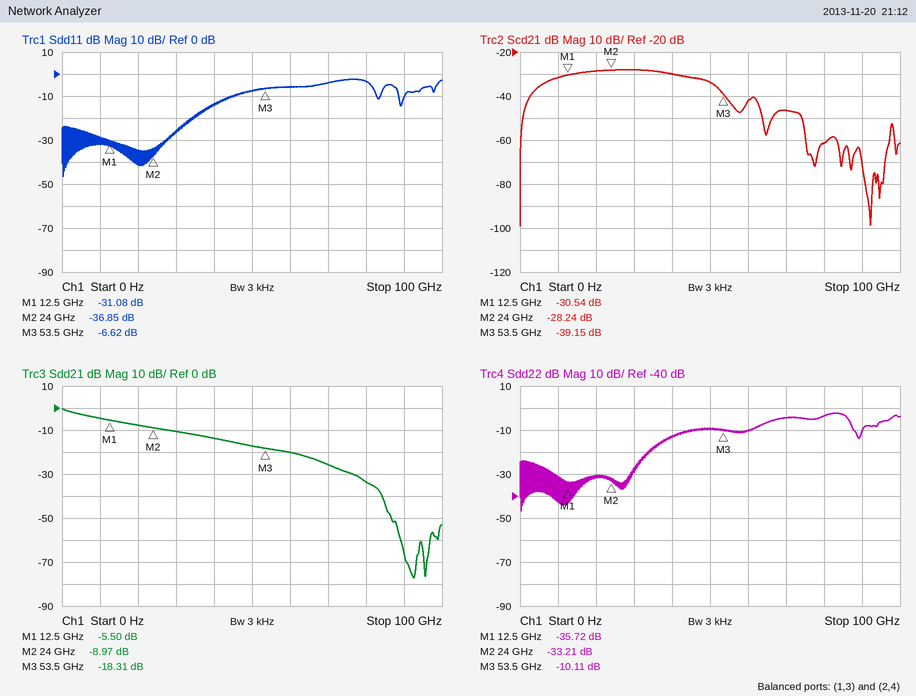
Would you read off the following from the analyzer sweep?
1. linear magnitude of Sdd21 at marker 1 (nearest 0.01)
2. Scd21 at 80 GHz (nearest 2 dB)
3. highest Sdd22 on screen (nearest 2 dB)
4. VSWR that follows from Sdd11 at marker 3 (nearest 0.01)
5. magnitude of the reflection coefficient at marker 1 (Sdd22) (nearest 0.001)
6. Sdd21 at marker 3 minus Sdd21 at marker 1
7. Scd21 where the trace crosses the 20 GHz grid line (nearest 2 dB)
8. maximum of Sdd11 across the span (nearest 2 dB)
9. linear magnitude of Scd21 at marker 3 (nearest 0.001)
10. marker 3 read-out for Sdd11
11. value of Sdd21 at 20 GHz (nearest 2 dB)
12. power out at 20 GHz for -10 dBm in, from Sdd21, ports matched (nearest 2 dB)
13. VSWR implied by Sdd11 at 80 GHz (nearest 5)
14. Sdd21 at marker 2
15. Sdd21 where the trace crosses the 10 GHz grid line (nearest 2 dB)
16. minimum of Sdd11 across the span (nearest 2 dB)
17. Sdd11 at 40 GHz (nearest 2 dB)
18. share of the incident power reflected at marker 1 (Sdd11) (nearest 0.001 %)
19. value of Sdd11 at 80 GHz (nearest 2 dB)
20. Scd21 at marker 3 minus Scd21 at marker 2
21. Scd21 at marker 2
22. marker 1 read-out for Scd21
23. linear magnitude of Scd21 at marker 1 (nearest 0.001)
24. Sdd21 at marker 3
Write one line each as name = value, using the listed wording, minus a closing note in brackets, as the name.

linear magnitude of Sdd21 at marker 1 = 0.53
Scd21 at 80 GHz = -62 dB
highest Sdd22 on screen = -2 dB
VSWR that follows from Sdd11 at marker 3 = 2.75
magnitude of the reflection coefficient at marker 1 (Sdd22) = 0.016
Sdd21 at marker 3 minus Sdd21 at marker 1 = -12.81 dB
Scd21 where the trace crosses the 20 GHz grid line = -28 dB
maximum of Sdd11 across the span = -2 dB
linear magnitude of Scd21 at marker 3 = 0.011
marker 3 read-out for Sdd11 = -6.62 dB
value of Sdd21 at 20 GHz = -8 dB
power out at 20 GHz for -10 dBm in, from Sdd21, ports matched = -18 dBm
VSWR implied by Sdd11 at 80 GHz = 5
Sdd21 at marker 2 = -8.97 dB
Sdd21 where the trace crosses the 10 GHz grid line = -4 dB
minimum of Sdd11 across the span = -46 dB
Sdd11 at 40 GHz = -14 dB
share of the incident power reflected at marker 1 (Sdd11) = 0.078 %
value of Sdd11 at 80 GHz = -4 dB
Scd21 at marker 3 minus Scd21 at marker 2 = -10.91 dB
Scd21 at marker 2 = -28.24 dB
marker 1 read-out for Scd21 = -30.54 dB
linear magnitude of Scd21 at marker 1 = 0.030
Sdd21 at marker 3 = -18.31 dB
